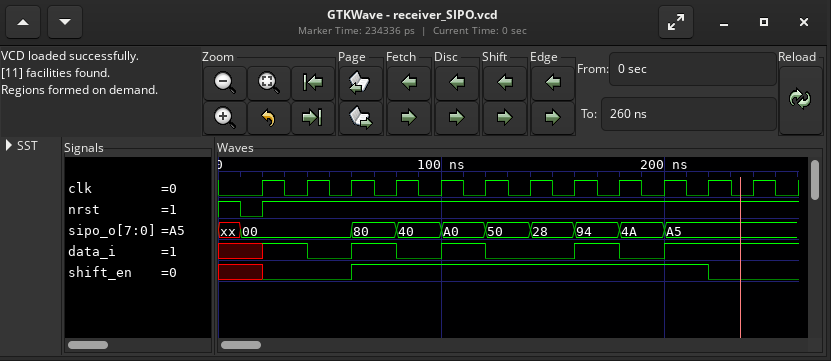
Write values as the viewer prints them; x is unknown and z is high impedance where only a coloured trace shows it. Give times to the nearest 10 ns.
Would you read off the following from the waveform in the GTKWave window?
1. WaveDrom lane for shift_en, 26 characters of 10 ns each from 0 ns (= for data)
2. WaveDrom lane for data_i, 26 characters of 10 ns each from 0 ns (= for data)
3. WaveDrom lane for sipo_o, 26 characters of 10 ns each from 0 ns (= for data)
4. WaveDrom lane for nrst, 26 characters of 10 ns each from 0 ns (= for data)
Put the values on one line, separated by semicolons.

{name: 'shift_en', wave: 'x.0...1...............0...'}; {name: 'data_i', wave: 'x.1.0.1.0.1.0...1.0.1.....'}; {name: 'sipo_o', wave: 'x=....=.=.=.=.=.=.=.=.....', data: '00 80 40 A0 50 28 94 4A A5'}; {name: 'nrst', wave: '101.......................'}
